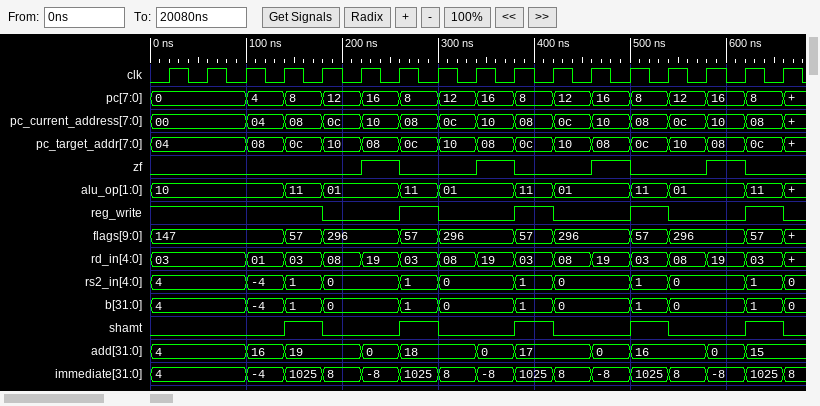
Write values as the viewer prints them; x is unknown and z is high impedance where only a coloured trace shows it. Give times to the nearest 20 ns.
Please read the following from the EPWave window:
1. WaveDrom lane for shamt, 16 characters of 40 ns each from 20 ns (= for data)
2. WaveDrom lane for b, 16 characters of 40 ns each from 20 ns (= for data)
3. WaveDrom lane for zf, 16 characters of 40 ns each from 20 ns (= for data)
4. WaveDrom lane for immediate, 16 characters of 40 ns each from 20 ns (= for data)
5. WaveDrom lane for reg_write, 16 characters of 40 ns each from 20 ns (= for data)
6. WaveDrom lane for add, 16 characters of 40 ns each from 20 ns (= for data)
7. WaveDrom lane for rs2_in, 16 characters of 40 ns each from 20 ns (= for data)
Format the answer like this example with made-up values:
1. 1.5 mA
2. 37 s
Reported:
1. {name: 'shamt', wave: '0..10.10.10.10.1'}
2. {name: 'b', wave: '=.===.==.==.==.=', data: '4 -4 1 0 1 0 1 0 1 0 1'}
3. {name: 'zf', wave: '0....10.10.10.10'}
4. {name: 'immediate', wave: '=.==============', data: '4 -4 1025 8 -8 1025 8 -8 1025 8 -8 1025 8 -8 1025'}
5. {name: 'reg_write', wave: '1...0.10.10.10.1'}
6. {name: 'add', wave: '=.==.==.==.==.==', data: '4 16 19 0 18 0 17 0 16 0 15'}
7. {name: 'rs2_in', wave: '=.===.==.==.==.=', data: '4 -4 1 0 1 0 1 0 1 0 1'}
